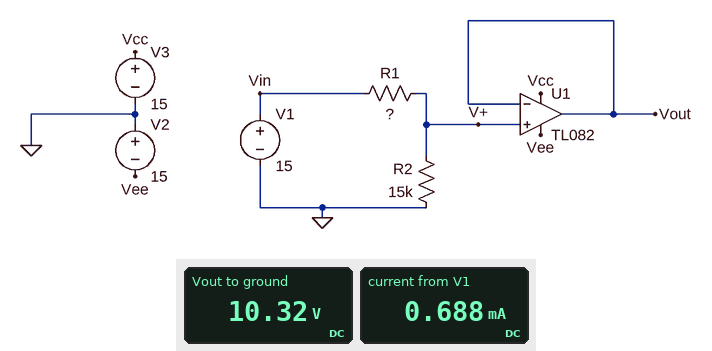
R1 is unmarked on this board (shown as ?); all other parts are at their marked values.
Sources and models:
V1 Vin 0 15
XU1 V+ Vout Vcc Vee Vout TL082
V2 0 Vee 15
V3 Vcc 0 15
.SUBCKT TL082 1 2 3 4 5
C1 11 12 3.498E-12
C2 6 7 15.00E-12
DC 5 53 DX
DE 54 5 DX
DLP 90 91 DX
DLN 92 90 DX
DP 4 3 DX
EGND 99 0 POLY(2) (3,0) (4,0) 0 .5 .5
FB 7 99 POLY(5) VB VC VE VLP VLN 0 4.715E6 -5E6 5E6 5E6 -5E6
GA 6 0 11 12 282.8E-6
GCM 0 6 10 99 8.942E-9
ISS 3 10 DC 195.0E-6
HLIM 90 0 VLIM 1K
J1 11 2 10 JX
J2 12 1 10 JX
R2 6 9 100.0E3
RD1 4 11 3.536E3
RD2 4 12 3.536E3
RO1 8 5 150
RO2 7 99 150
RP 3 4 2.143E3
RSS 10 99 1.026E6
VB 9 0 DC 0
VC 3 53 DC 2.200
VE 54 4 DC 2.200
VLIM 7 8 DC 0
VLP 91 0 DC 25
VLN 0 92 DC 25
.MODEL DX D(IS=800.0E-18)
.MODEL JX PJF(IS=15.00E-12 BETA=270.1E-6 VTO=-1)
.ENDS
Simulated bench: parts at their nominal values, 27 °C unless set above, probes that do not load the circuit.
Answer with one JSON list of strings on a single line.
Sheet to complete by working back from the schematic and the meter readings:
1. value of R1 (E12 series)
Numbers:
["6.8 kΩ"]
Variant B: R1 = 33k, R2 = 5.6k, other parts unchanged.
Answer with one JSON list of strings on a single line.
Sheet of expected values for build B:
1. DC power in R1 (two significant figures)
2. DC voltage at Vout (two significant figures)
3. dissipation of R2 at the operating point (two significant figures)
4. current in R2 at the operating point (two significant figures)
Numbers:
["5.0 mW", "2.2 V", "850 µW", "390 µA"]
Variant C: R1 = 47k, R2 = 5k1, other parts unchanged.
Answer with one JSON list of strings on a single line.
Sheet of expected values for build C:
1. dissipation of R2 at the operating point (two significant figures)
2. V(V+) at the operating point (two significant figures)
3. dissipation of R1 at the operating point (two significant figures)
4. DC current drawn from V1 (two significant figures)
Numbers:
["420 µW", "1.5 V", "3.9 mW", "290 µA"]
